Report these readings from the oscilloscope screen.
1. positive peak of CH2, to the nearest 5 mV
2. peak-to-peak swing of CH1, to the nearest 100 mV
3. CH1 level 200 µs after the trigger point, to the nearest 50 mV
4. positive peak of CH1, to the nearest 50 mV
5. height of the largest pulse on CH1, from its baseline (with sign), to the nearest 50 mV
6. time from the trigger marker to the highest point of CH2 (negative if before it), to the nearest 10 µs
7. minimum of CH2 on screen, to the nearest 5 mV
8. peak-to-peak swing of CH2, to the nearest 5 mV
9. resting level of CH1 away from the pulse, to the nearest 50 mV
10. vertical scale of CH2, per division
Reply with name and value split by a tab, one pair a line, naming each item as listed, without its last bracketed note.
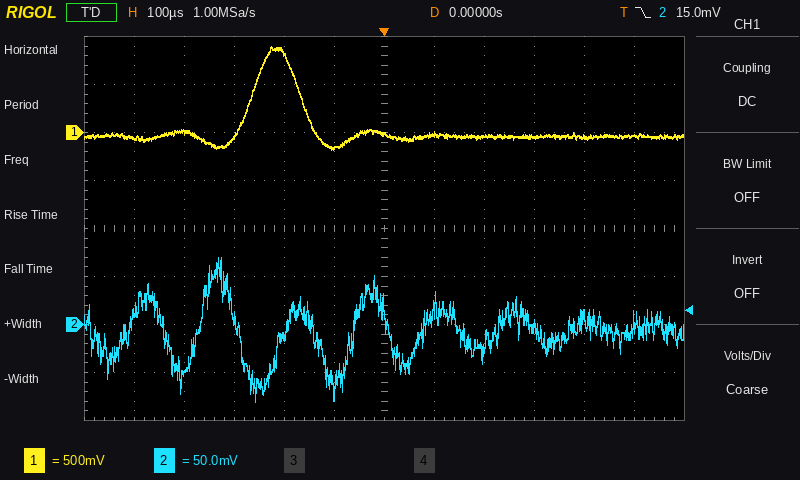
positive peak of CH2, to the nearest 5 mV	70 mV
peak-to-peak swing of CH1, to the nearest 100 mV	1.10 V
CH1 level 200 µs after the trigger point, to the nearest 50 mV	-50 mV
positive peak of CH1, to the nearest 50 mV	900 mV
height of the largest pulse on CH1, from its baseline (with sign), to the nearest 50 mV	+950 mV
time from the trigger marker to the highest point of CH2 (negative if before it), to the nearest 10 µs	-330 µs
minimum of CH2 on screen, to the nearest 5 mV	-80 mV
peak-to-peak swing of CH2, to the nearest 5 mV	150 mV
resting level of CH1 away from the pulse, to the nearest 50 mV	-50 mV
vertical scale of CH2, per division	50 mV
